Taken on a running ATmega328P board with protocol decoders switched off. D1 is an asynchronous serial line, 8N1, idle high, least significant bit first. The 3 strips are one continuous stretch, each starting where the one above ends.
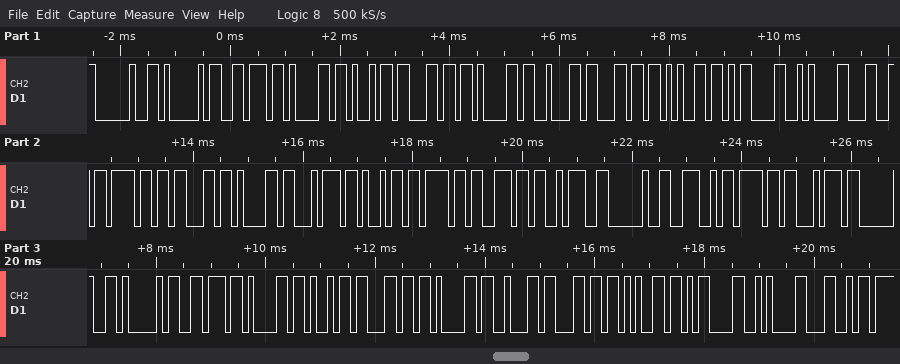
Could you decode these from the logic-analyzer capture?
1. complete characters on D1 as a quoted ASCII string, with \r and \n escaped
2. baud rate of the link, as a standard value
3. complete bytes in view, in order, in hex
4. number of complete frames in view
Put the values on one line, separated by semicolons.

" Available\r\nLocation: Not Available\r\nL"; 9600 baud; 0x20 0x41 0x76 0x61 0x69 0x6C 0x61 0x62 0x6C 0x65 0x0D 0x0A 0x4C 0x6F 0x63 0x61 0x74 0x69 0x6F 0x6E 0x3A 0x20 0x4E 0x6F 0x74 0x20 0x41 0x76 0x61 0x69 0x6C 0x61 0x62 0x6C 0x65 0x0D 0x0A 0x4C; 38
